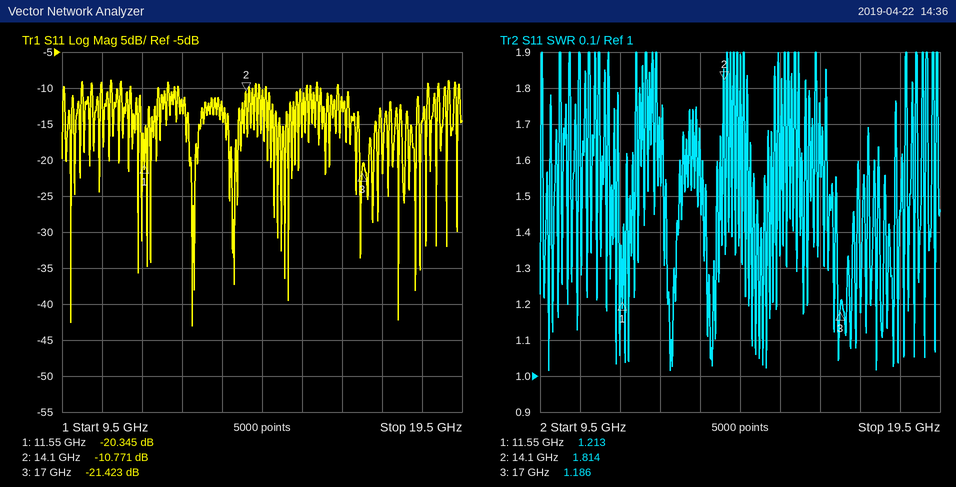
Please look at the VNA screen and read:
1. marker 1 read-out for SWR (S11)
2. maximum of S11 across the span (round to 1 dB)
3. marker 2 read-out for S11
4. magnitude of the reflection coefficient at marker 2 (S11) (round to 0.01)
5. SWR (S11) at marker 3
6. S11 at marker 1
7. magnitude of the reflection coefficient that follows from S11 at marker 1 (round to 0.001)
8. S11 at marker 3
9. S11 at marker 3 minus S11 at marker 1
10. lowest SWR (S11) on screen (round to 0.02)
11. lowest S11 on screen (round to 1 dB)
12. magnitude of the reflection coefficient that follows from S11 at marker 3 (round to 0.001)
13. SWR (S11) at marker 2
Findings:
1.213
-9 dB
-10.771 dB
0.29
1.186
-20.345 dB
0.096
-21.423 dB
-1.078 dB
1.02
-43 dB
0.085
1.814
